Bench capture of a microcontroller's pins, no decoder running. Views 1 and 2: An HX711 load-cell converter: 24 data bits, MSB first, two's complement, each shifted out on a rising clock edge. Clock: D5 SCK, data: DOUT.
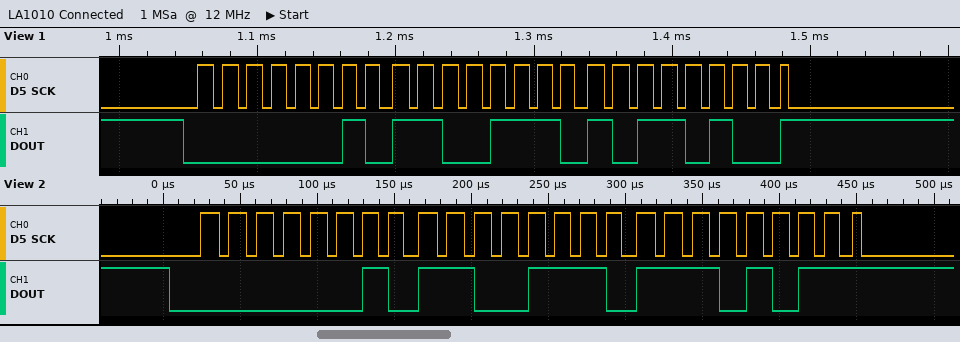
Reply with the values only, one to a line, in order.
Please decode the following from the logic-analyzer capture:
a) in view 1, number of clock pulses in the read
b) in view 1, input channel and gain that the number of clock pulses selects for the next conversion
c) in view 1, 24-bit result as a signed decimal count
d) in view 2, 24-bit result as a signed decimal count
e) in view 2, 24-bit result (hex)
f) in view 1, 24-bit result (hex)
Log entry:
25
channel A, gain 128
183988
184043
0x02CEEB
0x02CEB4
